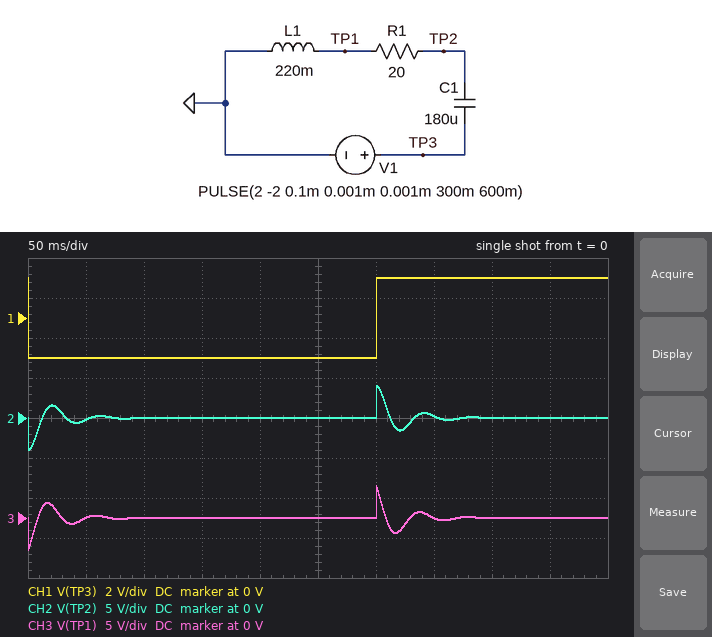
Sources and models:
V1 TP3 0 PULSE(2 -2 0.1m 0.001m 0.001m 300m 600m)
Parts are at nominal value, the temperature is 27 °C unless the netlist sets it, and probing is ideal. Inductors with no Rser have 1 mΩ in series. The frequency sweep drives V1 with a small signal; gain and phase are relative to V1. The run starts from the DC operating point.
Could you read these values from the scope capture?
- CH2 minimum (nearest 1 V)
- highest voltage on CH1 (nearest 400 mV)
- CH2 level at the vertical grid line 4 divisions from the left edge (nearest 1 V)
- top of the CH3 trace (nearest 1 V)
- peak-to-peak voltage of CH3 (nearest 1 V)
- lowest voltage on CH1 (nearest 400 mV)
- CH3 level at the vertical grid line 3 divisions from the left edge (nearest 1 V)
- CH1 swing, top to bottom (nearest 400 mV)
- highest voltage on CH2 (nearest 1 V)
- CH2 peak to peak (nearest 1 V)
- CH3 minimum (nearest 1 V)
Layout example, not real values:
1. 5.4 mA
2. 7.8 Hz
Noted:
1. -4 V
2. 2.0 V
3. 0 V
4. 4 V
5. 8 V
6. -2.0 V
7. 0 V
8. 4.0 V
9. 4 V
10. 8 V
11. -4 V
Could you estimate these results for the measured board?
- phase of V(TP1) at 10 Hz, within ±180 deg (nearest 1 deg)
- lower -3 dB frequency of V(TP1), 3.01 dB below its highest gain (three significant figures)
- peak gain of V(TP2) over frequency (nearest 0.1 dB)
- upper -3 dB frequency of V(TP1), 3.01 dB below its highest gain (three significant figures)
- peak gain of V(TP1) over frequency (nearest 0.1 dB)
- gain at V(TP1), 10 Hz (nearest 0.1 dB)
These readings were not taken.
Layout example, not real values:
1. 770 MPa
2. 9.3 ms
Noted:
1. 165 deg
2. 21.5 Hz
3. 6.3 dB
4. 47.1 Hz
5. 5.2 dB
6. -14.9 dB
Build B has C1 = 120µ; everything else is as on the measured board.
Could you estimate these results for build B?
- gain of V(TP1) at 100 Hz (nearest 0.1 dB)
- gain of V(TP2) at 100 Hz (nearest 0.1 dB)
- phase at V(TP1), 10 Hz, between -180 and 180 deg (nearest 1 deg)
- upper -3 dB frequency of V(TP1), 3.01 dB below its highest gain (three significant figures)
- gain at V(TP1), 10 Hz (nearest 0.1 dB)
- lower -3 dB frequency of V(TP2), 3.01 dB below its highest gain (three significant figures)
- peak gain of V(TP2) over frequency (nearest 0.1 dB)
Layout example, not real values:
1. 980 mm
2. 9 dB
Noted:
1. 0.8 dB
2. 0.9 dB
3. 170 deg
4. 46.9 Hz
5. -18.8 dB
6. 26.3 Hz
7. 7.6 dB
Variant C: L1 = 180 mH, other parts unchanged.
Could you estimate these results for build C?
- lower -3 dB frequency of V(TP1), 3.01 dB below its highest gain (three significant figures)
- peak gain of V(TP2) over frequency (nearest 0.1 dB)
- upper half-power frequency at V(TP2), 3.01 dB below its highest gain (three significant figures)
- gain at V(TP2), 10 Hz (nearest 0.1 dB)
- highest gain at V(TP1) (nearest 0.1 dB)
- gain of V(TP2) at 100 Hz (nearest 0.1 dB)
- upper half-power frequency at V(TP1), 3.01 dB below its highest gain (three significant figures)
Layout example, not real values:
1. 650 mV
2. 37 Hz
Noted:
1. 23.6 Hz
2. 5.7 dB
3. 50.8 Hz
4. -10.8 dB
5. 4.4 dB
6. 0.7 dB
7. 62.5 Hz
